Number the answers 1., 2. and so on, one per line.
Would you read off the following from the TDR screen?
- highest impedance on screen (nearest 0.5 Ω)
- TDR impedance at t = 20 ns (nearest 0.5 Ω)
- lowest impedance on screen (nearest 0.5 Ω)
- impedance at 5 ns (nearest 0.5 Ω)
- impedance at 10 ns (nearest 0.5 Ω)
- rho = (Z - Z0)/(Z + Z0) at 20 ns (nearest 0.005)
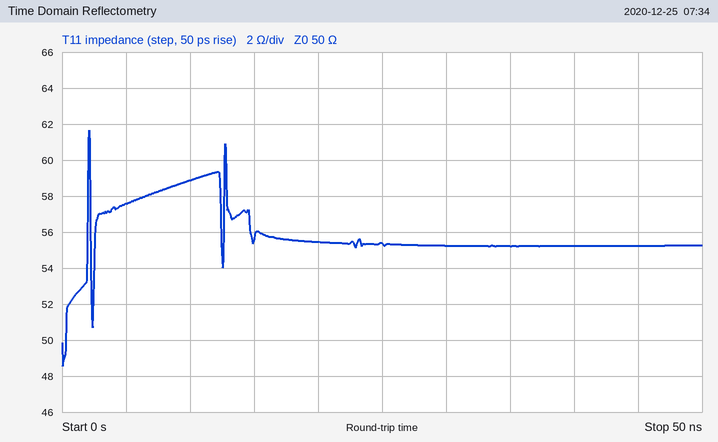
1. 61.5 Ω
2. 55.5 Ω
3. 48.5 Ω
4. 57.5 Ω
5. 59.0 Ω
6. +0.050
